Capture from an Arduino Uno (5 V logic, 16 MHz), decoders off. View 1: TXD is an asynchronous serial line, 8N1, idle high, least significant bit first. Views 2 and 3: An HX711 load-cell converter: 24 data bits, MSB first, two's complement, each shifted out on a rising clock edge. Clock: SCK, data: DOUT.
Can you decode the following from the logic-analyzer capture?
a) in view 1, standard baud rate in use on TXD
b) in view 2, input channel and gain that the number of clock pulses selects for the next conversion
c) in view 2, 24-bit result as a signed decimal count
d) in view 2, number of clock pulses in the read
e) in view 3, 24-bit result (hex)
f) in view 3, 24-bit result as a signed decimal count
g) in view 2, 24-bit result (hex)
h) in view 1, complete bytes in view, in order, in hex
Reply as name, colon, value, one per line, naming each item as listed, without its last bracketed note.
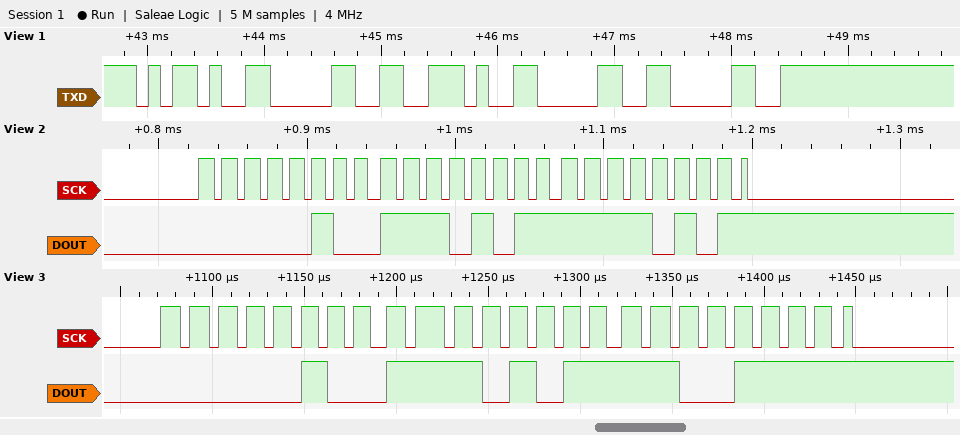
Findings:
in view 1, standard baud rate in use on TXD: 9600 baud
in view 2, input channel and gain that the number of clock pulses selects for the next conversion: channel A, gain 128
in view 2, 24-bit result as a signed decimal count: 322549
in view 2, number of clock pulses in the read: 25
in view 3, 24-bit result: 0x04EBCF
in view 3, 24-bit result as a signed decimal count: 322511
in view 2, 24-bit result: 0x04EBF5
in view 1, complete bytes in view, in order, in hex: 2D 30 2E 30 30
